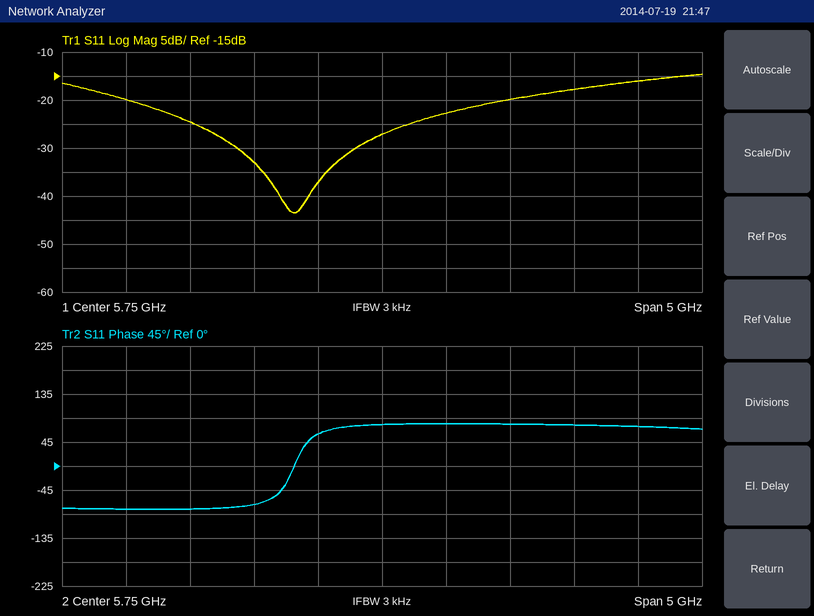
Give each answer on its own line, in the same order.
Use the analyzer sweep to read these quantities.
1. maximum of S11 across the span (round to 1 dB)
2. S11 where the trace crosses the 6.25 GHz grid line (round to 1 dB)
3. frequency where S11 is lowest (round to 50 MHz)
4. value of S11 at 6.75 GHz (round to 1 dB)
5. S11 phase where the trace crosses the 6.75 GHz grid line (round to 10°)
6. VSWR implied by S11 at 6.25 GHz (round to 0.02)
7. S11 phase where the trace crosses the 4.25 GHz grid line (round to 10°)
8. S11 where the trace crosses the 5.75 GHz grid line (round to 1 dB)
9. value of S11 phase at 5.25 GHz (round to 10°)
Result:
-15 dB
-23 dB
5.05 GHz
-20 dB
80°
1.16
-80°
-27 dB
60°
